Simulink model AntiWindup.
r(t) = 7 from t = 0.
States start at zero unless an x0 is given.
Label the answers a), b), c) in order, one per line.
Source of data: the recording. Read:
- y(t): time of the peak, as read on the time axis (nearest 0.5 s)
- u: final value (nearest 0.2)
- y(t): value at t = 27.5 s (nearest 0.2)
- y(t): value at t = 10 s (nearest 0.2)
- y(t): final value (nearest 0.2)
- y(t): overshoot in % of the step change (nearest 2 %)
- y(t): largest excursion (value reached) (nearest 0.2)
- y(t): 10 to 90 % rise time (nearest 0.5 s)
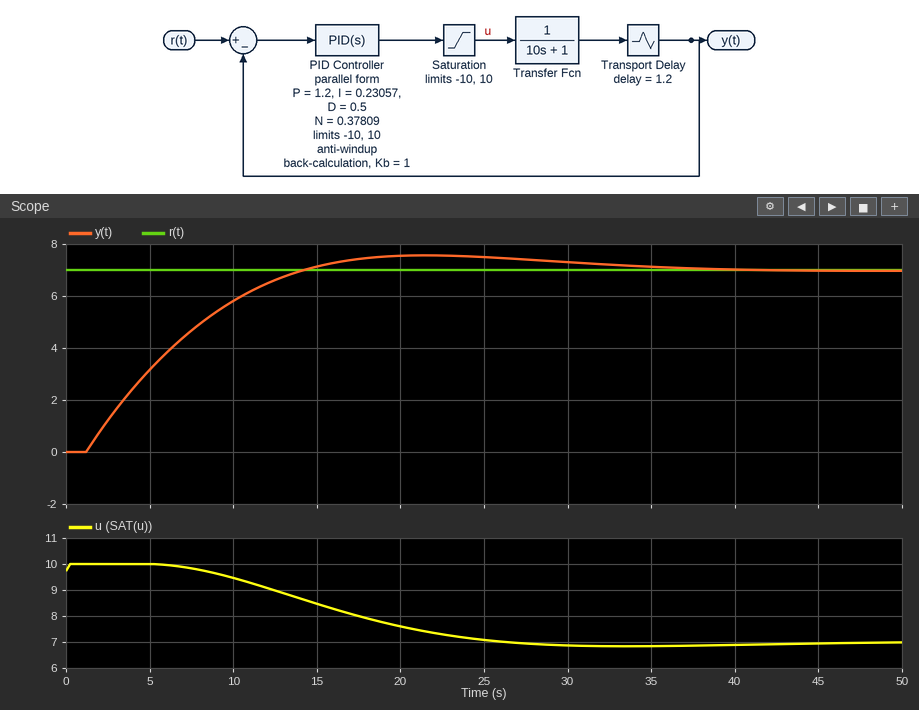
a) 21.5 s
b) 7.0
c) 7.4
d) 5.8
e) 7.0
f) 8 %
g) 7.6
h) 9.5 s
